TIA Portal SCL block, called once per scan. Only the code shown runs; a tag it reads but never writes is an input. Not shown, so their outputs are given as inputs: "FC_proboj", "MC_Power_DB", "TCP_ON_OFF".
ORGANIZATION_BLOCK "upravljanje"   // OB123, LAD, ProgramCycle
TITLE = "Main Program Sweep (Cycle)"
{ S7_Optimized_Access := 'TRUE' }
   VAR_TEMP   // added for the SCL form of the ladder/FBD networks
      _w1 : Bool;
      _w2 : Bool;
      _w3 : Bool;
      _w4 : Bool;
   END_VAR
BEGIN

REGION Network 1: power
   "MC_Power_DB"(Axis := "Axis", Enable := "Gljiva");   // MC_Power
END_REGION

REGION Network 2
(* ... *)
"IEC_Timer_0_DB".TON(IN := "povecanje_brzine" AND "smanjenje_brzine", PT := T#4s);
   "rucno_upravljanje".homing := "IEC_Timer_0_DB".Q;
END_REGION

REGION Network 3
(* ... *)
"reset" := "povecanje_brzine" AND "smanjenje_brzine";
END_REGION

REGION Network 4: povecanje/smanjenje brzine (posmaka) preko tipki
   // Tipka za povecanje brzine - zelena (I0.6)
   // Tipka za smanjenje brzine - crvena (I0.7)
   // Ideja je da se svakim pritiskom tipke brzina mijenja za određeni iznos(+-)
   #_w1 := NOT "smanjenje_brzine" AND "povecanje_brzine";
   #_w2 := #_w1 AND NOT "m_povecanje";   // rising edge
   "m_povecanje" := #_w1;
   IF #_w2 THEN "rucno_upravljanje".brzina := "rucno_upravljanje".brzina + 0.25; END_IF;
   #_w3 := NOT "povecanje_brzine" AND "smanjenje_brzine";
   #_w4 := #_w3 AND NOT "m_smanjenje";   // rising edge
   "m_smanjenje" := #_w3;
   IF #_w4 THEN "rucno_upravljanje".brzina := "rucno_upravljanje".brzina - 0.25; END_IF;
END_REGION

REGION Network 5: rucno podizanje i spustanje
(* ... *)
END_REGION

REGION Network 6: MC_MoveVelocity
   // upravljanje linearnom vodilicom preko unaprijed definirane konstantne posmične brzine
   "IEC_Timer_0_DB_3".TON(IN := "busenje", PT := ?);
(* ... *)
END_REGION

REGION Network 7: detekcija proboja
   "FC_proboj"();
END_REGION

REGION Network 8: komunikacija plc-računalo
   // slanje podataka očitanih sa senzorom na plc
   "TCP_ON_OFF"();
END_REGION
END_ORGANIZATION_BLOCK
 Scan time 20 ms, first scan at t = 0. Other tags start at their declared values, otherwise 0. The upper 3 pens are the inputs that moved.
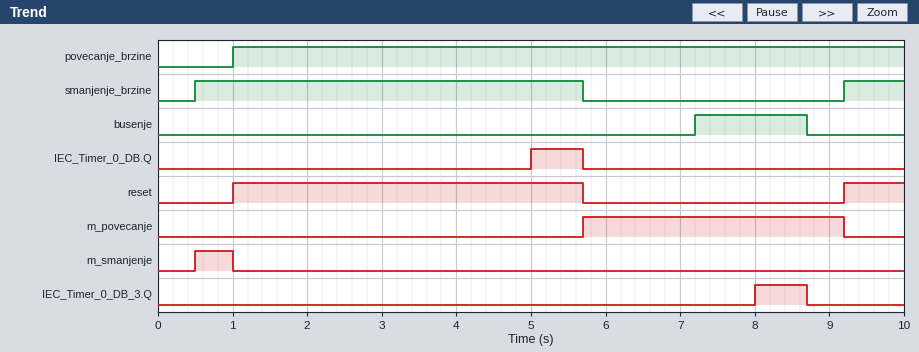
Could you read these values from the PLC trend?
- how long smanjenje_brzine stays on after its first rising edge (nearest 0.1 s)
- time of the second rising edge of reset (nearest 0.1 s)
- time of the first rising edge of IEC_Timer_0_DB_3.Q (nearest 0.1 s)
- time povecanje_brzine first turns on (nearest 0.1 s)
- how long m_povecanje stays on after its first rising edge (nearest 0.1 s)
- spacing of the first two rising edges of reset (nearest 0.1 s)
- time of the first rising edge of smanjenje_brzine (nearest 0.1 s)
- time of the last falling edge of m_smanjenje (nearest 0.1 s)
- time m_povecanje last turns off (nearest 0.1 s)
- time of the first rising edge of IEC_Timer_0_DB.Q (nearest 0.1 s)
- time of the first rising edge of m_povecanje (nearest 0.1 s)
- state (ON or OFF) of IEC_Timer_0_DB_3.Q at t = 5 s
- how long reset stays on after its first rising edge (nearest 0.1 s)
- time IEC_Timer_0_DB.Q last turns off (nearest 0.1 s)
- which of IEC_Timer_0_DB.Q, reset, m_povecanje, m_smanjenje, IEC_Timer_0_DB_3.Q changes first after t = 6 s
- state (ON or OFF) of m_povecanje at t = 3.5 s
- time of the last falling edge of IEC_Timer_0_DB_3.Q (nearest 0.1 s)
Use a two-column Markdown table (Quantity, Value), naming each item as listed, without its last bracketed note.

| Quantity | Value |
|---|---|
| how long smanjenje_brzine stays on after its first rising edge | 5.2 s |
| time of the second rising edge of reset | 9.2 s |
| time of the first rising edge of IEC_Timer_0_DB_3.Q | 8.0 s |
| time povecanje_brzine first turns on | 1.0 s |
| how long m_povecanje stays on after its first rising edge | 3.5 s |
| spacing of the first two rising edges of reset | 8.2 s |
| time of the first rising edge of smanjenje_brzine | 0.5 s |
| time of the last falling edge of m_smanjenje | 1.0 s |
| time m_povecanje last turns off | 9.2 s |
| time of the first rising edge of IEC_Timer_0_DB.Q | 5.0 s |
| time of the first rising edge of m_povecanje | 5.7 s |
| state (ON or OFF) of IEC_Timer_0_DB_3.Q at t = 5 s | OFF |
| how long reset stays on after its first rising edge | 4.7 s |
| time IEC_Timer_0_DB.Q last turns off | 5.7 s |
| which of IEC_Timer_0_DB.Q, reset, m_povecanje, m_smanjenje, IEC_Timer_0_DB_3.Q changes first after t = 6 s | IEC_Timer_0_DB_3.Q |
| state (ON or OFF) of m_povecanje at t = 3.5 s | OFF |
| time of the last falling edge of IEC_Timer_0_DB_3.Q | 8.7 s |
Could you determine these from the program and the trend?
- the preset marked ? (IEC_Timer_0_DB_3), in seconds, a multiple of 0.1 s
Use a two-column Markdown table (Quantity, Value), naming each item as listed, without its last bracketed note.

| Quantity | Value |
|---|---|
| the preset marked ? (IEC_Timer_0_DB_3), in seconds, a multiple of 0.1 s | 0.8 s |
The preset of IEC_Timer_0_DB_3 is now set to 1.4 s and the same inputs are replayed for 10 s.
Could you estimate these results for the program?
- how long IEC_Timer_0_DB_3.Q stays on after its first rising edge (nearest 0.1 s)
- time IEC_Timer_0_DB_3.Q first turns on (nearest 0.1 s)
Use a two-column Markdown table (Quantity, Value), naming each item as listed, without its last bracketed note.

| Quantity | Value |
|---|---|
| how long IEC_Timer_0_DB_3.Q stays on after its first rising edge | 0.1 s |
| time IEC_Timer_0_DB_3.Q first turns on | 8.6 s |
